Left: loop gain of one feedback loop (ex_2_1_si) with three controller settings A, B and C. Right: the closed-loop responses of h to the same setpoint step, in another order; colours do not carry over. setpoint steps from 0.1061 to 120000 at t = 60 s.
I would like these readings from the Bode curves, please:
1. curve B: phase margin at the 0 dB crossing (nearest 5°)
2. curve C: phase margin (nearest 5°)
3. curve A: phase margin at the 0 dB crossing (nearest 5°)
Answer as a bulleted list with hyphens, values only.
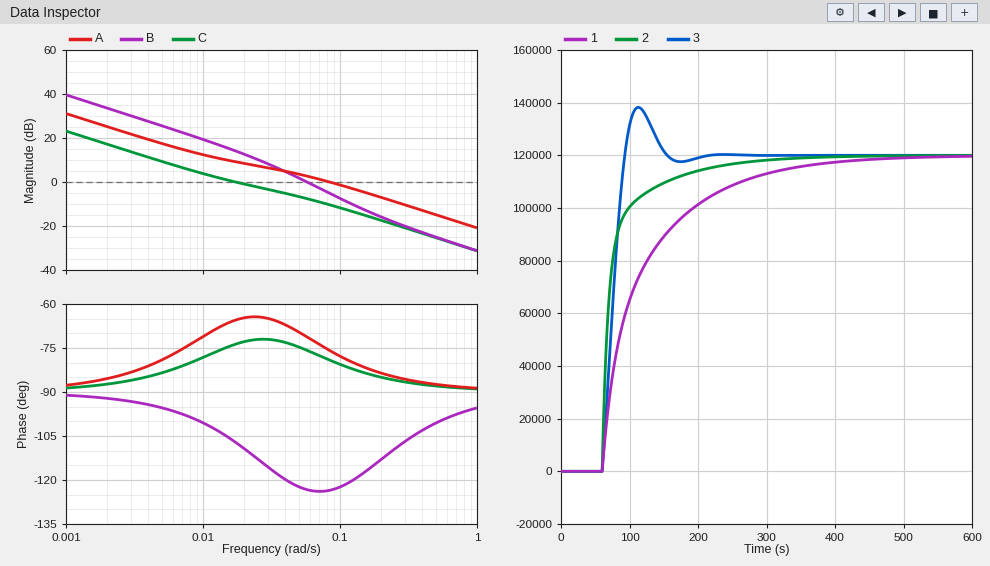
- 55°
- 105°
- 105°
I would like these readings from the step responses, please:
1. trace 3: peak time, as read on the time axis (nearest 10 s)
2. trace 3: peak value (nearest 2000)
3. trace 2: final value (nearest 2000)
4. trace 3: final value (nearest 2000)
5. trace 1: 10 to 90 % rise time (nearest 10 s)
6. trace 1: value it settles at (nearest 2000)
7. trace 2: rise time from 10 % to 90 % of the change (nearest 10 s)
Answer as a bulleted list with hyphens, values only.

- 110 s
- 138000
- 120000
- 120000
- 180 s
- 120000
- 80 s
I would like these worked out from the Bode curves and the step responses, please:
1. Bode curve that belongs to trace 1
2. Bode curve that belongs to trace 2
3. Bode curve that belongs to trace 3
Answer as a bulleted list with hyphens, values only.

- C
- A
- B
